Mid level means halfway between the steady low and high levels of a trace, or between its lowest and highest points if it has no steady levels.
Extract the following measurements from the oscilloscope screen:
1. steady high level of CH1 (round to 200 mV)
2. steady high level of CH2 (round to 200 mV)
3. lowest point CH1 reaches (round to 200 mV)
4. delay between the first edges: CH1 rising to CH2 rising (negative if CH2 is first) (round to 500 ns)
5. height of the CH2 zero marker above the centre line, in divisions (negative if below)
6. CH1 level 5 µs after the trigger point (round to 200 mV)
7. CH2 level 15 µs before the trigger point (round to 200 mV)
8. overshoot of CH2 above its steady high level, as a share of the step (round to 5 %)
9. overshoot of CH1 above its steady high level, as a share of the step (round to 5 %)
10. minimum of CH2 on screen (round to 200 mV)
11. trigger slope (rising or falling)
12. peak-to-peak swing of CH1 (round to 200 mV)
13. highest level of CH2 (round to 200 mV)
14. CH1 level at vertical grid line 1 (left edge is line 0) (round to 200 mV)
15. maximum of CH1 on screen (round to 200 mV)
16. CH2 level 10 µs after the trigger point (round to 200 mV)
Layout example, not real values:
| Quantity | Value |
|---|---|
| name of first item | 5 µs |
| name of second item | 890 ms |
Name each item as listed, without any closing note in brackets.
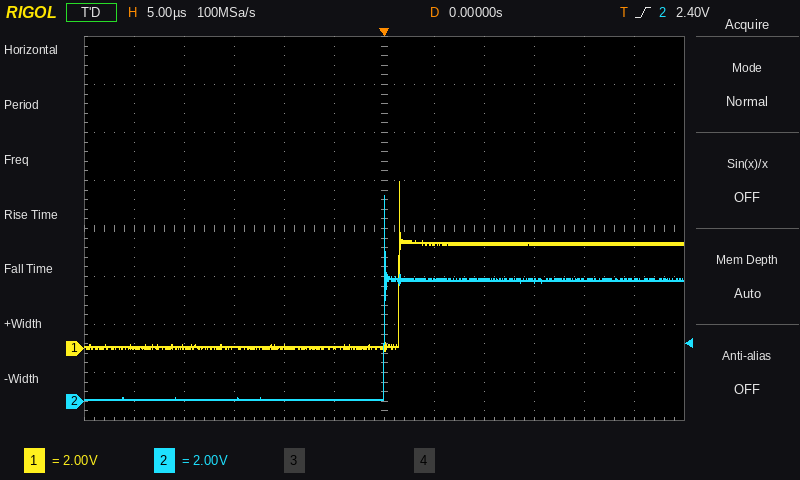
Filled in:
| Quantity | Value |
|---|---|
| steady high level of CH1 | 4.4 V |
| steady high level of CH2 | 5.0 V |
| lowest point CH1 reaches | 0.0 V |
| delay between the first edges: CH1 rising to CH2 rising (negative if CH2 is first) | -1.5 µs |
| height of the CH2 zero marker above the centre line, in divisions | -3.6 div |
| CH1 level 5 µs after the trigger point | 4.4 V |
| CH2 level 15 µs before the trigger point | 0.0 V |
| overshoot of CH2 above its steady high level, as a share of the step | 70 % |
| overshoot of CH1 above its steady high level, as a share of the step | 60 % |
| minimum of CH2 on screen | 0.0 V |
| trigger slope | rising |
| peak-to-peak swing of CH1 | 7.0 V |
| highest level of CH2 | 8.6 V |
| CH1 level at vertical grid line 1 (left edge is line 0) | 0.0 V |
| maximum of CH1 on screen | 7.0 V |
| CH2 level 10 µs after the trigger point | 5.0 V |
